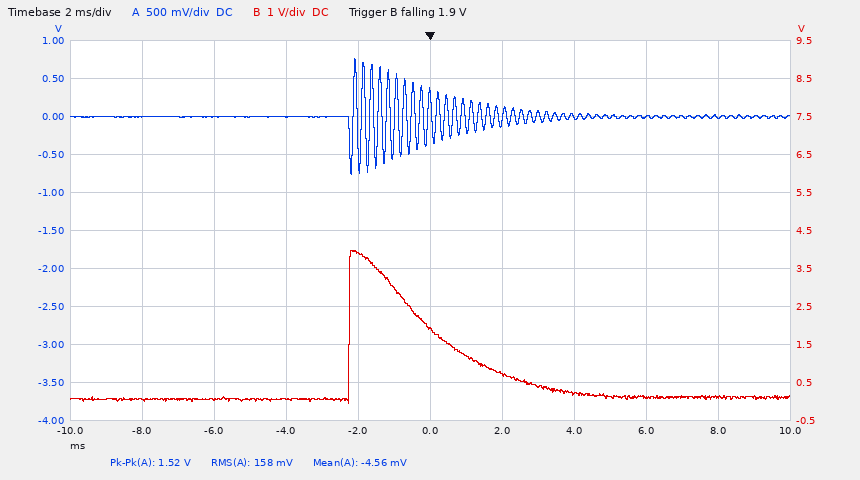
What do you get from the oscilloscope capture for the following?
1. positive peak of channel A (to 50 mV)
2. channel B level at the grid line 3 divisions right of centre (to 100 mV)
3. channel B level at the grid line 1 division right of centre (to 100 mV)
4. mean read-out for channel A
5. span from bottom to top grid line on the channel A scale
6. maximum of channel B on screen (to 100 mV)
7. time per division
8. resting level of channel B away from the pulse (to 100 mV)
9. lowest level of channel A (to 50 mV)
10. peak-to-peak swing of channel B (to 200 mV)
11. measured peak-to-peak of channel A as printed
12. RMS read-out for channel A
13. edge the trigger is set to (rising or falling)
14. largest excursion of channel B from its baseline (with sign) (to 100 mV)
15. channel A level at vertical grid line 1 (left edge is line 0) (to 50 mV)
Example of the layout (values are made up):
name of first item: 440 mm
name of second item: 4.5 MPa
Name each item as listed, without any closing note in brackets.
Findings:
positive peak of channel A: 750 mV
channel B level at the grid line 3 divisions right of centre: 100 mV
channel B level at the grid line 1 division right of centre: 700 mV
mean read-out for channel A: -4.56 mV
span from bottom to top grid line on the channel A scale: 5 V
maximum of channel B on screen: 4.0 V
time per division: 2 ms
resting level of channel B away from the pulse: 100 mV
lowest level of channel A: -750 mV
peak-to-peak swing of channel B: 4.0 V
measured peak-to-peak of channel A as printed: 1.52 V
RMS read-out for channel A: 158 mV
edge the trigger is set to: falling
largest excursion of channel B from its baseline (with sign): +3.9 V
channel A level at vertical grid line 1 (left edge is line 0): 0 mV
